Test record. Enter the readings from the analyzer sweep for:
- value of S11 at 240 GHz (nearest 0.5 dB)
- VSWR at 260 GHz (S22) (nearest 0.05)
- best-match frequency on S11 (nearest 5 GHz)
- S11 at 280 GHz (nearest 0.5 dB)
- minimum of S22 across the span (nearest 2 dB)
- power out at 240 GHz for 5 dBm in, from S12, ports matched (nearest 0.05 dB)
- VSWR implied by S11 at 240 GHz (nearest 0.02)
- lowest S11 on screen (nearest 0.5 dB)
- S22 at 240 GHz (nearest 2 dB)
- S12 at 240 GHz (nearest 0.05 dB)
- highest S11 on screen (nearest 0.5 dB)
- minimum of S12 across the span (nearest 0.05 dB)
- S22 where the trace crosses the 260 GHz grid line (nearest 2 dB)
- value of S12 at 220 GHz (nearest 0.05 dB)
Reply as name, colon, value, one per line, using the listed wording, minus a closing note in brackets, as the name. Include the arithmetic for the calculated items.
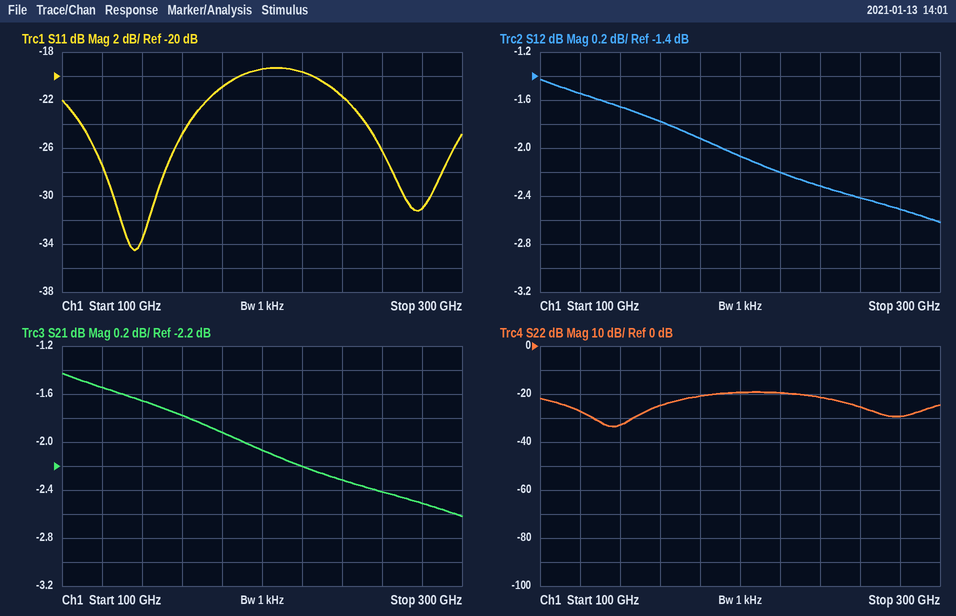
value of S11 at 240 GHz: -21.5 dB
VSWR at 260 GHz (S22): |Γ| = 10^(-26/20) = 0.0501; VSWR = (1 + 0.0501)/(1 − 0.0501) ≈ 1.11, so 1.10 to the nearest 0.05
best-match frequency on S11: 135 GHz
S11 at 280 GHz: -31.0 dB
minimum of S22 across the span: -34 dB
power out at 240 GHz for 5 dBm in, from S12, ports matched: 5 dBm + (-2.30 dB) = 2.70 dBm
VSWR implied by S11 at 240 GHz: |Γ| = 10^(-21.5/20) = 0.0841; VSWR = (1 + 0.0841)/(1 − 0.0841) ≈ 1.18
lowest S11 on screen: -34.5 dB
S22 at 240 GHz: -22 dB
S12 at 240 GHz: -2.30 dB
highest S11 on screen: -19.5 dB
minimum of S12 across the span: -2.60 dB
S22 where the trace crosses the 260 GHz grid line: -26 dB
value of S12 at 220 GHz: -2.20 dB
